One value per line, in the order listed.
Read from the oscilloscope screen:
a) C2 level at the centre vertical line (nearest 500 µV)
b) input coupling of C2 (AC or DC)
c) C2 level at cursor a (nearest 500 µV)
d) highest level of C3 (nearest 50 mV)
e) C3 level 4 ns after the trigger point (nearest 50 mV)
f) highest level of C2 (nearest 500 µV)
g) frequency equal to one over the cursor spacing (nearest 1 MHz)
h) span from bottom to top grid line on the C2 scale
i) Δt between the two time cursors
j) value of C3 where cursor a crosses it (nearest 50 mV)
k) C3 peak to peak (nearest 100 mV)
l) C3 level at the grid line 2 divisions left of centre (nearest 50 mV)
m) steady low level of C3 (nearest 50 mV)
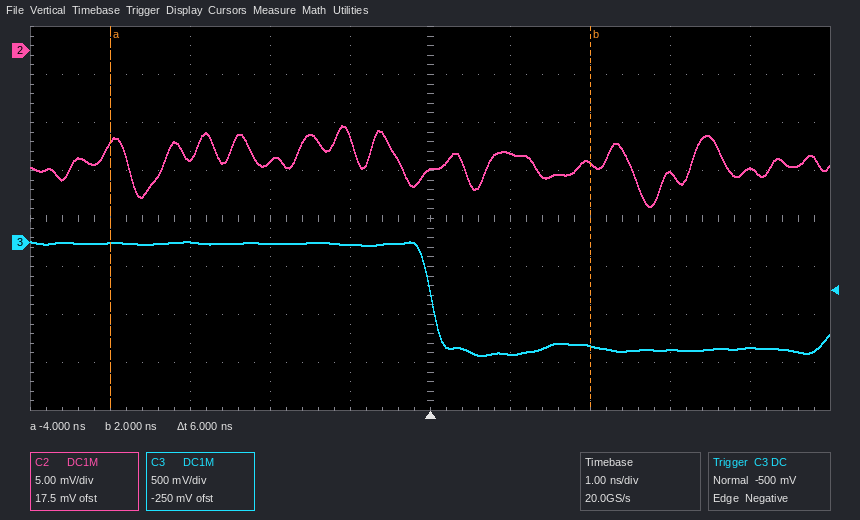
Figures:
-12.5 mV
DC
-9.5 mV
0 mV
-1.10 V
-8.0 mV
167 MHz
40 mV
6 ns
0 mV
1.20 V
0 mV
-1.10 V
